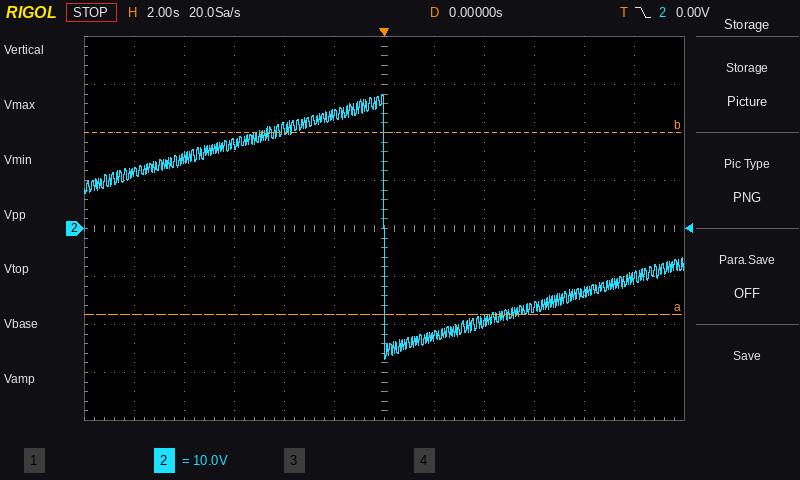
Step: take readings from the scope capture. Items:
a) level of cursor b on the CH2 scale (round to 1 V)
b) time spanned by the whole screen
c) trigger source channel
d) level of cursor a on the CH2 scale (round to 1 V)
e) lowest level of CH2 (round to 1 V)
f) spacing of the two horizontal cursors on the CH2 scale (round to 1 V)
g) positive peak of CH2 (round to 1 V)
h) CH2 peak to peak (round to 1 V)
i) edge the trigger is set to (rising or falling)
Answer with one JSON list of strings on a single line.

["20 V", "24 s", "CH2", "-18 V", "-27 V", "38 V", "28 V", "55 V", "falling"]
